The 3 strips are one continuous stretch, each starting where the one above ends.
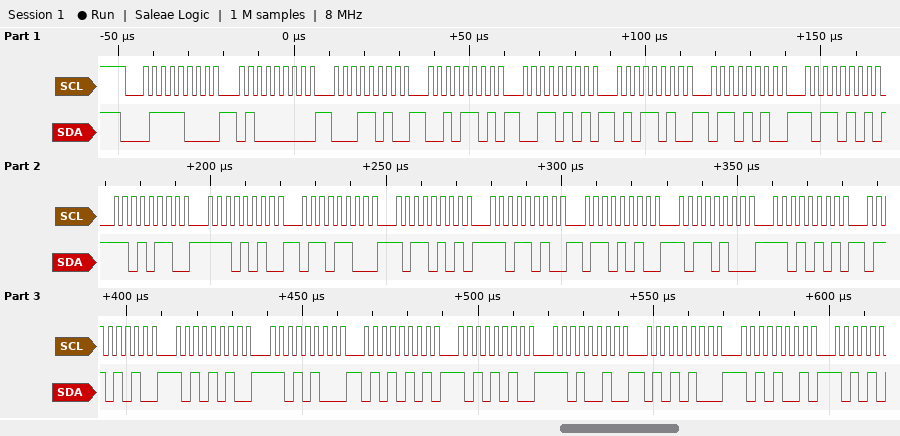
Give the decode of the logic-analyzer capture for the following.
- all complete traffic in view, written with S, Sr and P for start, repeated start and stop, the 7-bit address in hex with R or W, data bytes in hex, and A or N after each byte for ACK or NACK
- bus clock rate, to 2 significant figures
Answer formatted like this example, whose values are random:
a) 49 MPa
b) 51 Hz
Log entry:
a) S 3CW A 40 A 1A A 2D A 35 A 5A A 6A A B5 A D6 A EA A 6C A B5 A DA A 6A A B4 A D5 A 6A A AA A D4 A 55 A AA A D2 A 54 A A9 A
b) 400 kHz
